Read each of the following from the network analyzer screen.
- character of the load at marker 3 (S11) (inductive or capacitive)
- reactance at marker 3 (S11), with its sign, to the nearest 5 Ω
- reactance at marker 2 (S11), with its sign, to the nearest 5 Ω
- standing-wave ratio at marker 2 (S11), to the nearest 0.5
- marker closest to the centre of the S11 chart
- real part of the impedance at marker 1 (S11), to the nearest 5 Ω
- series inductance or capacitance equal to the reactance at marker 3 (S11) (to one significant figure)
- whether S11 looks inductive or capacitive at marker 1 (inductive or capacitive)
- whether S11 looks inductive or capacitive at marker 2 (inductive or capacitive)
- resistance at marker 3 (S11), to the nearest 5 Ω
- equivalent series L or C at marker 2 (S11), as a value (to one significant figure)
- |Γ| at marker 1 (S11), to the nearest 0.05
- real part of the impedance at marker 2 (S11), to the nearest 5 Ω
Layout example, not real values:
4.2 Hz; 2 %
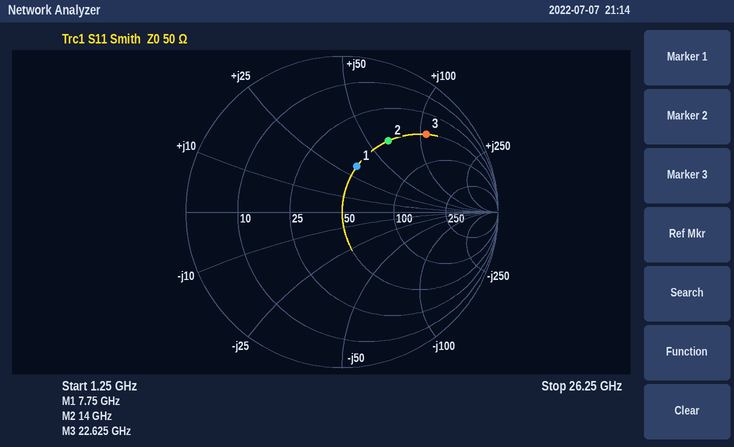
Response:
inductive; +110 Ω; +65 Ω; 3.5; marker 1; 50 Ω; 800 pH; inductive; inductive; 50 Ω; 700 pH; 0.30; 50 Ω
